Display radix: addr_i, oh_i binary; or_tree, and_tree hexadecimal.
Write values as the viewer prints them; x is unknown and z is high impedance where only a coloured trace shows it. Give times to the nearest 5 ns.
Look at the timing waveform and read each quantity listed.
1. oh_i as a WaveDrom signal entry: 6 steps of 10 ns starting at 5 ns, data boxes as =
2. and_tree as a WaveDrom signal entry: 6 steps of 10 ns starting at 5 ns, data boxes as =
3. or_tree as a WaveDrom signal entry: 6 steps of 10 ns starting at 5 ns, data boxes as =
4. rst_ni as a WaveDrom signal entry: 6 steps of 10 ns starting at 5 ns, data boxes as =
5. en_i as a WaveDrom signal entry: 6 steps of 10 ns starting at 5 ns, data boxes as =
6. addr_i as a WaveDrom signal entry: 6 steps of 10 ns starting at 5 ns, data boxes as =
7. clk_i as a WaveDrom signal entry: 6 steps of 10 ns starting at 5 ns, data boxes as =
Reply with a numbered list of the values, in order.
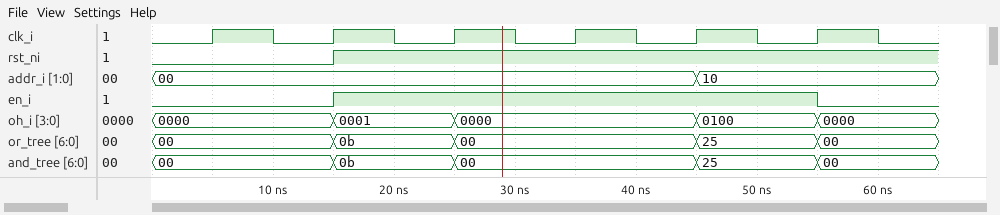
1. {name: 'oh_i', wave: '===.==', data: '0000 0001 0000 0100 0000'}
2. {name: 'and_tree', wave: '===.==', data: '00 0b 00 25 00'}
3. {name: 'or_tree', wave: '===.==', data: '00 0b 00 25 00'}
4. {name: 'rst_ni', wave: '01....'}
5. {name: 'en_i', wave: '01...0'}
6. {name: 'addr_i', wave: '=...=.', data: '00 10'}
7. {name: 'clk_i', wave: 'p.....'}
